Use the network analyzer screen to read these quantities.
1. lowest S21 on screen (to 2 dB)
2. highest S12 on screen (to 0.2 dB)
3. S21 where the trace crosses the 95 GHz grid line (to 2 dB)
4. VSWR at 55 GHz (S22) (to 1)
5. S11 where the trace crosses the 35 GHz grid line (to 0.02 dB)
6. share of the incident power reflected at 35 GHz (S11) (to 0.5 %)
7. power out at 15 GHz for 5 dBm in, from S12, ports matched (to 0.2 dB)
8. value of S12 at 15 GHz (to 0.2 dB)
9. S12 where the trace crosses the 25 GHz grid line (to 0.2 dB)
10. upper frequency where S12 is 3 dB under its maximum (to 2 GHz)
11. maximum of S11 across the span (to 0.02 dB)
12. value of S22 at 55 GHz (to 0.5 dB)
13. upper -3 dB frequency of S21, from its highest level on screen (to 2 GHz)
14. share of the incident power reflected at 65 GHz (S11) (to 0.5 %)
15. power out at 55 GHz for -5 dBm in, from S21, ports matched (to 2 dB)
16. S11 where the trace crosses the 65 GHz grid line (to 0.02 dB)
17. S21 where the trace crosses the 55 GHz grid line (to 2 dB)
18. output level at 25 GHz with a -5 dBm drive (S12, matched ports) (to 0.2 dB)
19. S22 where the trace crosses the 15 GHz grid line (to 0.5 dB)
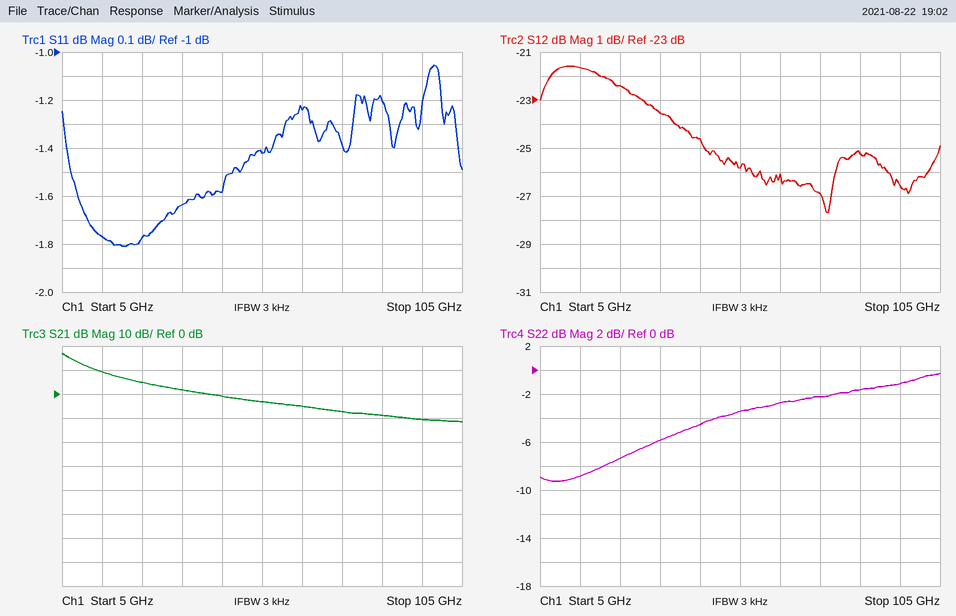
-12 dB
-21.6 dB
-10 dB
5
-1.64 dB
68.5 %
-16.6 dBm
-21.6 dB
-22.4 dB
44 GHz
-1.06 dB
-3.5 dB
8 GHz
75.0 %
-8 dBm
-1.24 dB
-4 dB
-27.4 dBm
-9.0 dB
